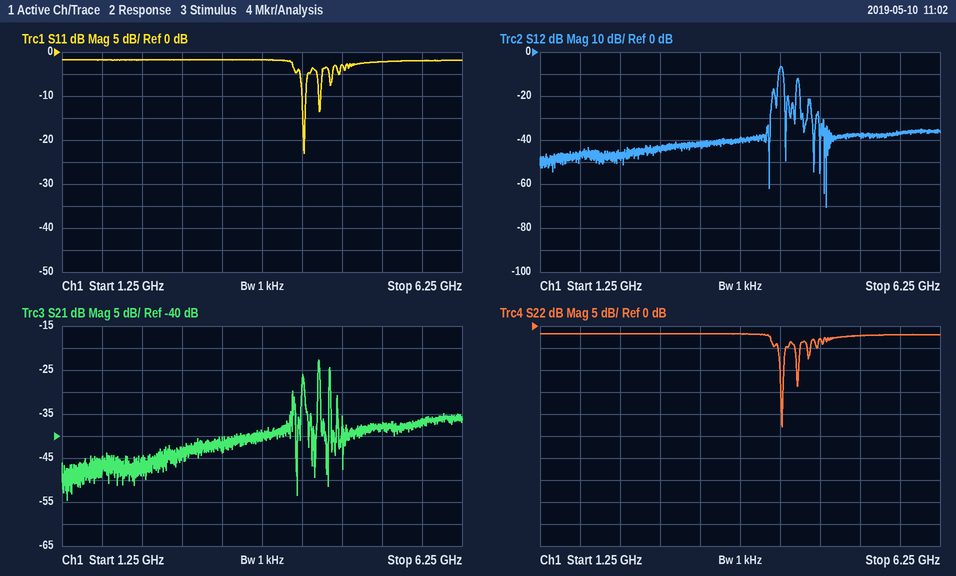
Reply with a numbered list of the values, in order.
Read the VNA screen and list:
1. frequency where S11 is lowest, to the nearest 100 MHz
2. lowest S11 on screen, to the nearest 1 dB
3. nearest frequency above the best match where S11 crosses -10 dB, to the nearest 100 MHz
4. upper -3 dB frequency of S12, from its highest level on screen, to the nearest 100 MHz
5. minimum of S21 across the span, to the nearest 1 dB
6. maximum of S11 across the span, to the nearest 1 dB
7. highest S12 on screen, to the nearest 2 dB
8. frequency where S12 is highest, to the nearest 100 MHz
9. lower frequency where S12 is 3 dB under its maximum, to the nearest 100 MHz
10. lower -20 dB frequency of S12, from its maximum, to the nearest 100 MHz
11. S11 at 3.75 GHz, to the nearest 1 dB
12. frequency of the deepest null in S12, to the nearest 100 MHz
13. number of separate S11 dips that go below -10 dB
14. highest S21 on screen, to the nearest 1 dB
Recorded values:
1. 4.3 GHz
2. -23 dB
3. 4.3 GHz
4. 4.3 GHz
5. -55 dB
6. -2 dB
7. -6 dB
8. 4.3 GHz
9. 4.2 GHz
10. 4.1 GHz
11. -2 dB
12. 4.8 GHz
13. 2
14. -23 dB
